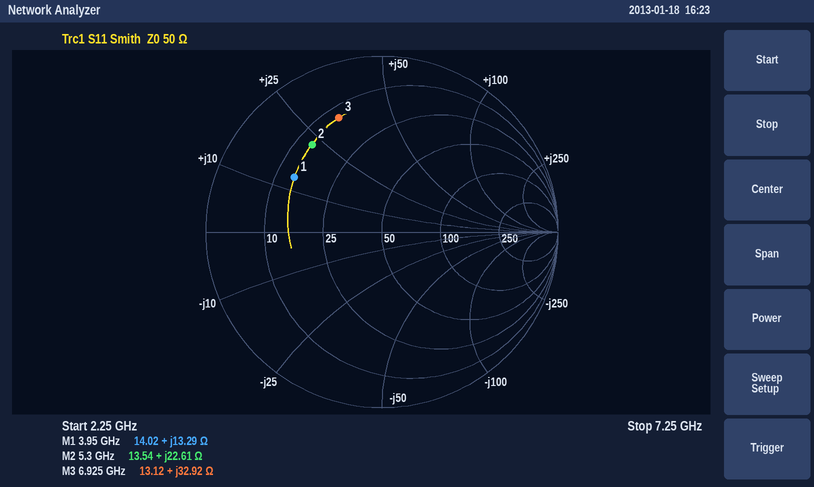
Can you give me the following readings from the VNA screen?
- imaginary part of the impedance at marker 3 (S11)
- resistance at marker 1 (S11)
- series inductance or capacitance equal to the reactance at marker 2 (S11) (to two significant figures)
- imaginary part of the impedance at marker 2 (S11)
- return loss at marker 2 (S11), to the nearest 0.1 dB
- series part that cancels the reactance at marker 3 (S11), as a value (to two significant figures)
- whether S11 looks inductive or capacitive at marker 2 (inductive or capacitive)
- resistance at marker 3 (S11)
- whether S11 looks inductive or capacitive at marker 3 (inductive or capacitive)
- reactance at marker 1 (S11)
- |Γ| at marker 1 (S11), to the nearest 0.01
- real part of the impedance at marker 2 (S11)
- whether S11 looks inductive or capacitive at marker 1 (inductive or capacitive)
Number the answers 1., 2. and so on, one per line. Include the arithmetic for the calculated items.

1. +32.92 Ω
2. 14.02 Ω
3. L = 22.61 Ω/(2π × 5.3 GHz) ≈ 679 pH, so 680 pH to two significant figures
4. +22.61 Ω
5. 3.9 dB
6. C = 1/(2π × 6.925 GHz × 32.92 Ω) ≈ 698 fF, so 700 fF to two significant figures
7. inductive
8. 13.12 Ω
9. inductive
10. +13.29 Ω
11. 0.59
12. 13.54 Ω
13. inductive
